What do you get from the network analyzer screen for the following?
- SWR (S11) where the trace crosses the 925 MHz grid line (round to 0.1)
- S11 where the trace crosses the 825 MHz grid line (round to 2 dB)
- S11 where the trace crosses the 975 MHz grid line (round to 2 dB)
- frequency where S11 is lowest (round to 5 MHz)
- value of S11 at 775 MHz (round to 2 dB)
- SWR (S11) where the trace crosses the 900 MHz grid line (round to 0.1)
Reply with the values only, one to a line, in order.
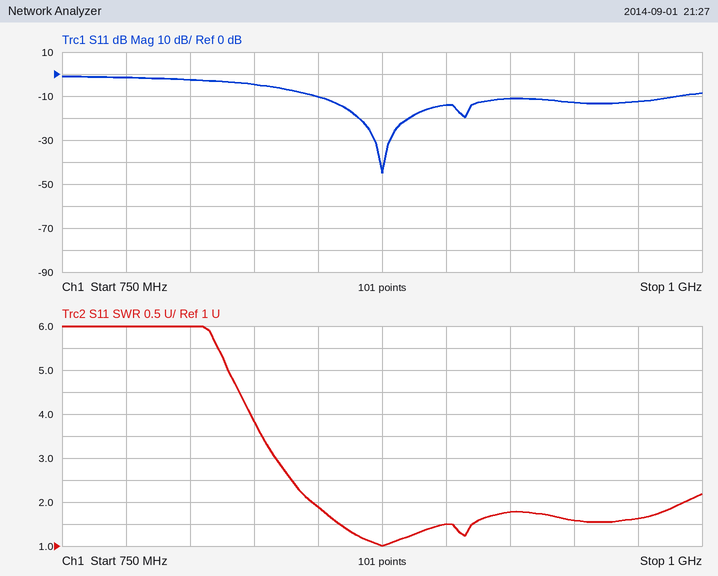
1.8
-4 dB
-12 dB
875 MHz
-2 dB
1.5
